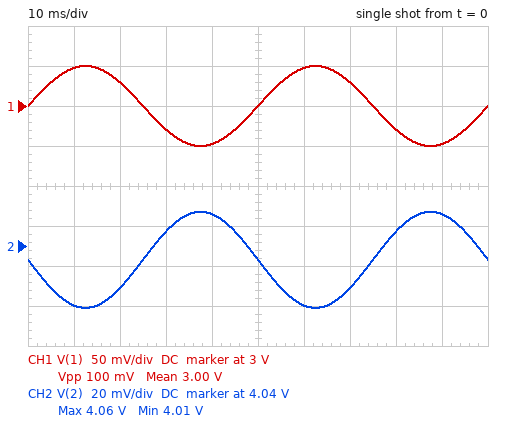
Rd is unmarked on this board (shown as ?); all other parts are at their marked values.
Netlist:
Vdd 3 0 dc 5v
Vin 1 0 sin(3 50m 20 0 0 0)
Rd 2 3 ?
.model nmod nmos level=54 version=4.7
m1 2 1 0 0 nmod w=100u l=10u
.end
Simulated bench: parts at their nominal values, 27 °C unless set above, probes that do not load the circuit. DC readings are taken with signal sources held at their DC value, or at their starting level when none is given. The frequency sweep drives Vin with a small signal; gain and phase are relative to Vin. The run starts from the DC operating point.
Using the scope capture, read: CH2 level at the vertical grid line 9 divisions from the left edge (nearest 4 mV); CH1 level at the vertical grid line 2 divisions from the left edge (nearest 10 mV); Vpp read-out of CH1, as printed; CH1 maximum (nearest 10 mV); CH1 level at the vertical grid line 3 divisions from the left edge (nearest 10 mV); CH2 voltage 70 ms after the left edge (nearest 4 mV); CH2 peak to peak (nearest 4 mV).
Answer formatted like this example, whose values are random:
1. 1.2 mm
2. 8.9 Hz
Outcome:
1. 4.056 V
2. 3.03 V
3. 100 mV
4. 3.05 V
5. 2.97 V
6. 4.020 V
7. 48 mV
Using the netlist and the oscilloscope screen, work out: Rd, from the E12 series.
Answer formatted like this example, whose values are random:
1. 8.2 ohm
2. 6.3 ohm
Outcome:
1. 82 Ω
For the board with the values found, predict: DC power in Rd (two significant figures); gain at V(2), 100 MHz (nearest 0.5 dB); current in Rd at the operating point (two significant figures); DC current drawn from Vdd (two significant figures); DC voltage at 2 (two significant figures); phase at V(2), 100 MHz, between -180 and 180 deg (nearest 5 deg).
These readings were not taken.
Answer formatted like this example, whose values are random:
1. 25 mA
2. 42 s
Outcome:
1. 11 mW
2. -6.0 dB
3. 12 mA
4. 12 mA
5. 4.0 V
6. 160 deg
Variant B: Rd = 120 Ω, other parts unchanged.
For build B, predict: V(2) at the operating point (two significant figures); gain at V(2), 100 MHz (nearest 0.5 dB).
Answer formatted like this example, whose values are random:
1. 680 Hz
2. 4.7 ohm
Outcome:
1. 3.6 V
2. -2.5 dB
